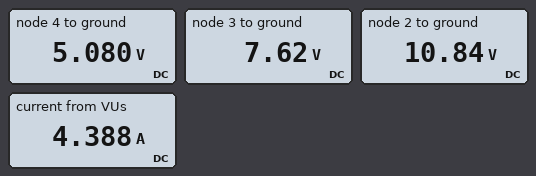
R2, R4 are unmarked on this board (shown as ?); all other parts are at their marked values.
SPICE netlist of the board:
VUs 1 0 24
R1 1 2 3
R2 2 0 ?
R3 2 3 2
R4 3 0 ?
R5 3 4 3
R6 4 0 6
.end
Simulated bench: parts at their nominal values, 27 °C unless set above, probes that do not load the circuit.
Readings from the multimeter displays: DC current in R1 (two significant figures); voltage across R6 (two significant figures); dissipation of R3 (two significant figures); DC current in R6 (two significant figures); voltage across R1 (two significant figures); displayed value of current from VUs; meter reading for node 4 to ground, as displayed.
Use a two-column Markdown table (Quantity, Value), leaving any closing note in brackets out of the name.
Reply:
| Quantity | Value |
|---|---|
| DC current in R1 | 4.4 A |
| voltage across R6 | 5.1 V |
| dissipation of R3 | 5.2 W |
| DC current in R6 | 850 mA |
| voltage across R1 | 13 V |
| displayed value of current from VUs | 4.388 A |
| meter reading for node 4 to ground, as displayed | 5.080 V |
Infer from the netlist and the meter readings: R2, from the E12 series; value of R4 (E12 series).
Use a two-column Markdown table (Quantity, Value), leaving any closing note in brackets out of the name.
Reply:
| Quantity | Value |
|---|---|
| R2, from the E12 series | 3.9 Ω |
| value of R4 | 10 Ω |
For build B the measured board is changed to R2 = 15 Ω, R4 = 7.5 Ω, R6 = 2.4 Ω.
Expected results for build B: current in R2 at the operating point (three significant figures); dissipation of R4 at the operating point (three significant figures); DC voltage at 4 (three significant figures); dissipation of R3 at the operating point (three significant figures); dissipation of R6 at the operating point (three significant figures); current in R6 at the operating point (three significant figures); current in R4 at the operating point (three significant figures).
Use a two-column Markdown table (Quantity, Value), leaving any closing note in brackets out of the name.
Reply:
| Quantity | Value |
|---|---|
| current in R2 at the operating point | 897 mA |
| dissipation of R4 at the operating point | 9.01 W |
| DC voltage at 4 | 3.65 V |
| dissipation of R3 at the operating point | 13.7 W |
| dissipation of R6 at the operating point | 5.56 W |
| current in R6 at the operating point | 1.52 A |
| current in R4 at the operating point | 1.10 A |
